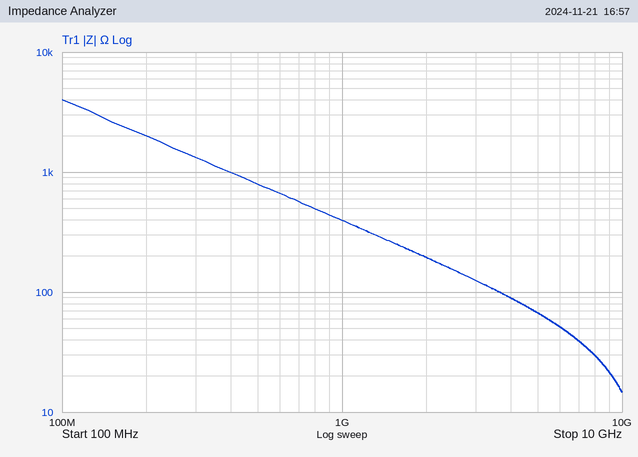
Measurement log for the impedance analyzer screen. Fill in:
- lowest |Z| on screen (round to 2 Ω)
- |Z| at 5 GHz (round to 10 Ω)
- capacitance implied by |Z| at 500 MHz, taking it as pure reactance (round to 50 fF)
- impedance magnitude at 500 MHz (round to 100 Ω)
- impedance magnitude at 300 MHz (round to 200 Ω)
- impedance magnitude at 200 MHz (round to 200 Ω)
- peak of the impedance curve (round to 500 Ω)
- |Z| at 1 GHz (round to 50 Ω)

14 Ω
70 Ω
400 fF
800 Ω
1.4 kΩ
2.0 kΩ
4.0 kΩ
400 Ω
